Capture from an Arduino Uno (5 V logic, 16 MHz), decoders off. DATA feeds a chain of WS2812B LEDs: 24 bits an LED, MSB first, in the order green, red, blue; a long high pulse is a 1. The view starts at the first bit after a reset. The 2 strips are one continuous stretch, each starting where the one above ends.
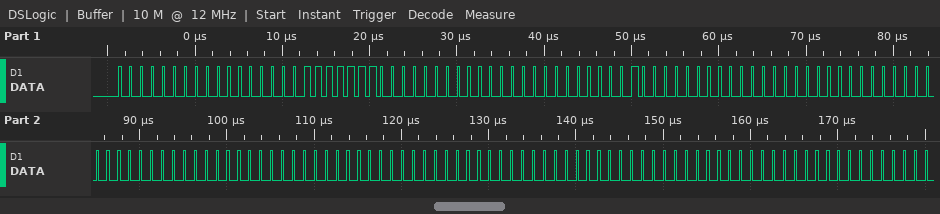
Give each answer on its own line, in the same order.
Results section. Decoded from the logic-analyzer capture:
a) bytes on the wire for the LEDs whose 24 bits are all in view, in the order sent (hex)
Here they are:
00 00 7F 00 00 01 00 00 00 00 00 00 00 00 00 00 00 00
